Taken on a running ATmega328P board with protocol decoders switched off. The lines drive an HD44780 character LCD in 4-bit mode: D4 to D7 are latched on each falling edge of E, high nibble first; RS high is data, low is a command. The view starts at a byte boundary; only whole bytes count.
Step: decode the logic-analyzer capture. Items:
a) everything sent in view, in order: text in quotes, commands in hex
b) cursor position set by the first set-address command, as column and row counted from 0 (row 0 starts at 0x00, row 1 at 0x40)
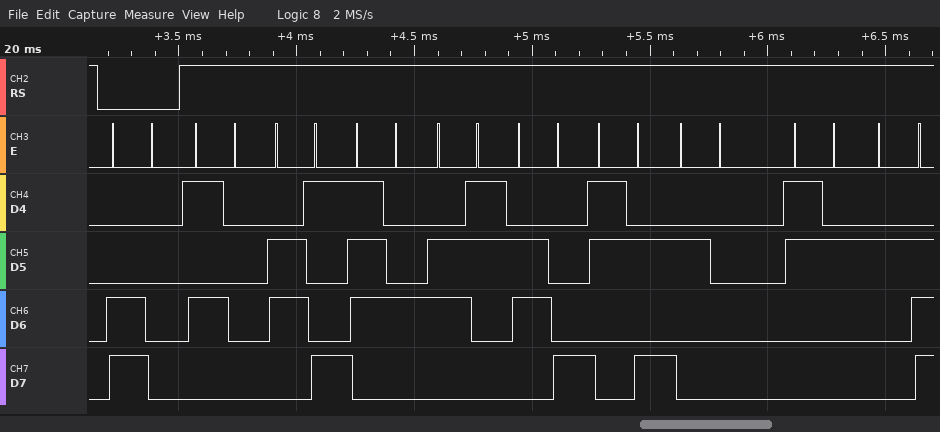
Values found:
0xC0 "Pitch: 2."
column 0, row 1
